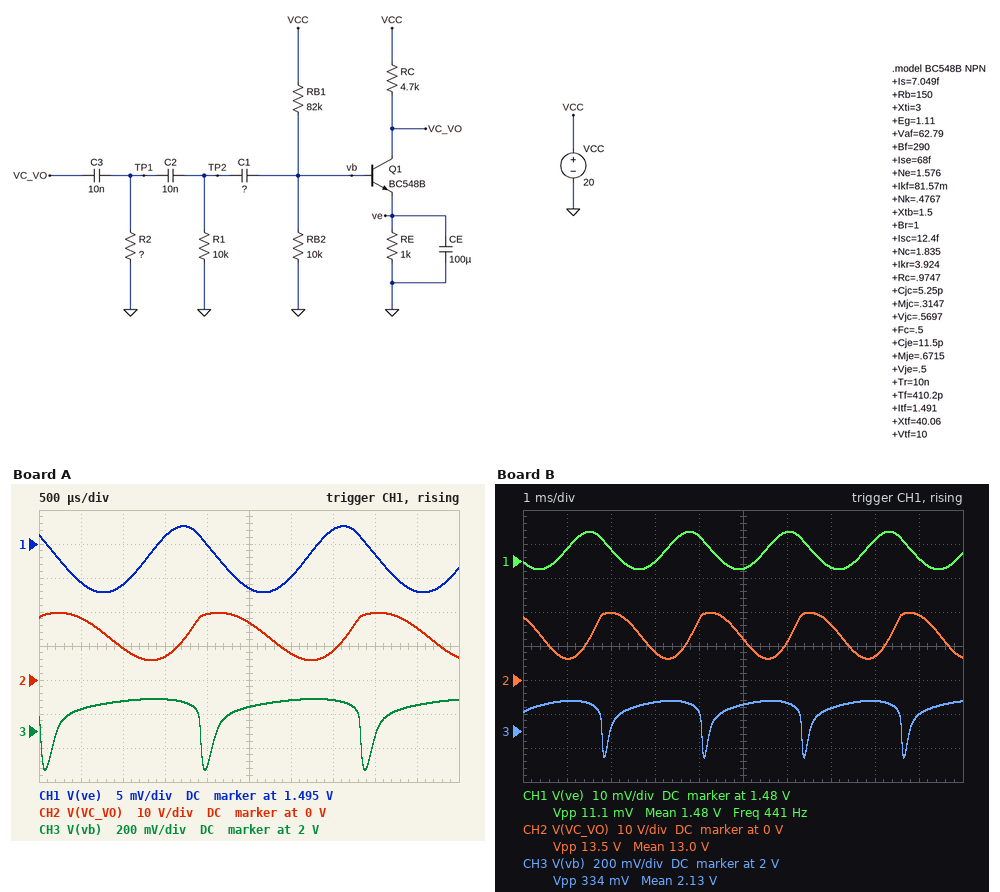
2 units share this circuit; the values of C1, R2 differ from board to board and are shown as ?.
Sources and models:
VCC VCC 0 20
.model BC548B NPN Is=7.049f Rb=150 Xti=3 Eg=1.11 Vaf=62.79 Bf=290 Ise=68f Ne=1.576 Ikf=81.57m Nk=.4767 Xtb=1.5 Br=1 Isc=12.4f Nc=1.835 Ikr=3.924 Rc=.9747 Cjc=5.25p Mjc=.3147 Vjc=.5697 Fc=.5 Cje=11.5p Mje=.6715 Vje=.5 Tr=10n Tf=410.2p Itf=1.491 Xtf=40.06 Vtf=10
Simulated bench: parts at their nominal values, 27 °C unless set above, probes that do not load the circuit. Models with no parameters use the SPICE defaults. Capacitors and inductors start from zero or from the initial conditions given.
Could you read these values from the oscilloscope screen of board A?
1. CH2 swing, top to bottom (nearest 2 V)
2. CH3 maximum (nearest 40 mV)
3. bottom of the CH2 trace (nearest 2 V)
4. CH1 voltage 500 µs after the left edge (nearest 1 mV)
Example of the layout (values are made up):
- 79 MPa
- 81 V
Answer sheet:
- 14 V
- 2.20 V
- 6 V
- 1.489 V
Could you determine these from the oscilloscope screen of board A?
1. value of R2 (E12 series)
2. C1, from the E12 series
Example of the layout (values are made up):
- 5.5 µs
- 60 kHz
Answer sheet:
- 8.2 kΩ
- 12 nF
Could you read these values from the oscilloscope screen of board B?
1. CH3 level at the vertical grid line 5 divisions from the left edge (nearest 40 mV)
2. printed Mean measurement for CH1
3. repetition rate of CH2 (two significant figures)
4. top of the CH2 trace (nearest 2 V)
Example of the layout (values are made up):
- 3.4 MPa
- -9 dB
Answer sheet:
- 2.16 V
- 1.48 V
- 440 Hz
- 20 V
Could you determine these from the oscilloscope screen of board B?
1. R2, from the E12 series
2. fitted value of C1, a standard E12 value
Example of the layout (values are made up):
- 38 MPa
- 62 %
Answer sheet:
- 22 kΩ
- 8.2 nF
